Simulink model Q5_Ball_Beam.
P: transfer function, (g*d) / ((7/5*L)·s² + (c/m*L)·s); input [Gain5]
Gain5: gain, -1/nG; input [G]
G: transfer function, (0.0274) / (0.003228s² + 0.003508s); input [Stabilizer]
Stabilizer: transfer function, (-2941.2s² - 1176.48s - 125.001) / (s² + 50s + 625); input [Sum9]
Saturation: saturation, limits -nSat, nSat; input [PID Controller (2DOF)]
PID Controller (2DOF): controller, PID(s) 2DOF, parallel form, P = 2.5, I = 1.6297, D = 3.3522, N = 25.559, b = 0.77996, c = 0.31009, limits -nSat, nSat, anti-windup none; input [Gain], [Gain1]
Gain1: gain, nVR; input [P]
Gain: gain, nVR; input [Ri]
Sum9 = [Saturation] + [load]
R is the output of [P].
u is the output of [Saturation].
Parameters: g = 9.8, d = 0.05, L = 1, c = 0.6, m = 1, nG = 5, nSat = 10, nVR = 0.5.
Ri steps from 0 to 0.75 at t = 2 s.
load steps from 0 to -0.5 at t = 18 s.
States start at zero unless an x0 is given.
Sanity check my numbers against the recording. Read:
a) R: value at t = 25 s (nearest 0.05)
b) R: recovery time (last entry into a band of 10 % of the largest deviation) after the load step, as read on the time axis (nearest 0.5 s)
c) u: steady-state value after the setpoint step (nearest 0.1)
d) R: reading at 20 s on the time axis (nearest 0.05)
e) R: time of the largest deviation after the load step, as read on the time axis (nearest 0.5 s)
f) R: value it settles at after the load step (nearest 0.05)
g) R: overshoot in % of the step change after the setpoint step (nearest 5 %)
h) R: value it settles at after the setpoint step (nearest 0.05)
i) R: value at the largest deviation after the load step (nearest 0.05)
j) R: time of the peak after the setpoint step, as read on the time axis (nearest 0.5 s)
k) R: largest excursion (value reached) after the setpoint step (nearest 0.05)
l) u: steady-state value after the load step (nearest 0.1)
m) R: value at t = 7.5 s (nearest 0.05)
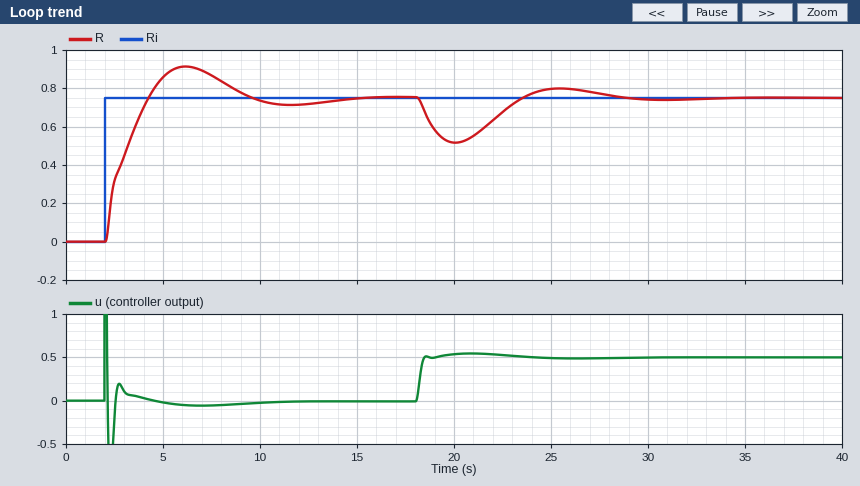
0.80
27.5 s
0.0
0.50
20.0 s
0.75
20 %
0.75
0.50
6.0 s
0.90
0.5
0.85
